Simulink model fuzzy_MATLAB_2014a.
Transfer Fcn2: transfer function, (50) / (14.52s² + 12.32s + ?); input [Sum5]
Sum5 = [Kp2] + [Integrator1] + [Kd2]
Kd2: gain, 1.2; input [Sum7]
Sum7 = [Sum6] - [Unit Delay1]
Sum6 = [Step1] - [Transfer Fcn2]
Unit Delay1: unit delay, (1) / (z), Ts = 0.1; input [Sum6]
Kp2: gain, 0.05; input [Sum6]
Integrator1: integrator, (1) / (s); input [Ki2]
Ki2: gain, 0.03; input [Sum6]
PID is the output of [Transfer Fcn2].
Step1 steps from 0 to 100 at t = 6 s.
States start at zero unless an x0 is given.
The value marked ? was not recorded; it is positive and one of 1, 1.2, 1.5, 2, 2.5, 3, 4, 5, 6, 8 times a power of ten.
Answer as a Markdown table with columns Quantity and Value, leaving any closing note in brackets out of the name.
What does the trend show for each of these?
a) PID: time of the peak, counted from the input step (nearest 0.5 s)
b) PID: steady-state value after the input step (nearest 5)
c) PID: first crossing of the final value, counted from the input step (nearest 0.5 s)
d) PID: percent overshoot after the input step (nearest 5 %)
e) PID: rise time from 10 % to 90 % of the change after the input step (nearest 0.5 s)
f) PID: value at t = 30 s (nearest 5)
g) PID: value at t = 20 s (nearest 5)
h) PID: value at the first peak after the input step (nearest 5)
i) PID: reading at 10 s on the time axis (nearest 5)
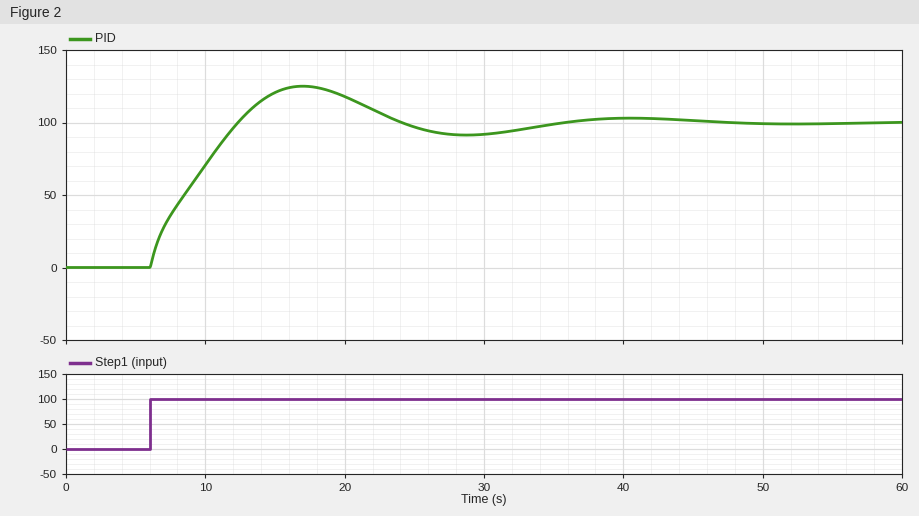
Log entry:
| Quantity | Value |
|---|---|
| PID: time of the peak, counted from the input step | 11.0 s |
| PID: steady-state value after the input step | 100 |
| PID: first crossing of the final value, counted from the input step | 6.5 s |
| PID: percent overshoot after the input step | 25 % |
| PID: rise time from 10 % to 90 % of the change after the input step | 5.0 s |
| PID: value at t = 30 s | 90 |
| PID: value at t = 20 s | 120 |
| PID: value at the first peak after the input step | 125 |
| PID: reading at 10 s on the time axis | 70 |
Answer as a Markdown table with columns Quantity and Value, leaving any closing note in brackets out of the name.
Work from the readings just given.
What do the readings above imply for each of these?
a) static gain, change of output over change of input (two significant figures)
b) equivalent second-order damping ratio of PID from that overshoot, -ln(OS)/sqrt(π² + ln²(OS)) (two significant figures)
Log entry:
| Quantity | Value |
|---|---|
| static gain, change of output over change of input | 1.0 |
| equivalent second-order damping ratio of PID from that overshoot, -ln(OS)/sqrt(π² + ln²(OS)) | 0.40 |
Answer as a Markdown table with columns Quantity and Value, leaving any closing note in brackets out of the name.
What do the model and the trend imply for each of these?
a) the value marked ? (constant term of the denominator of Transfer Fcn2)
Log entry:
| Quantity | Value |
|---|---|
| the value marked ? | 2 |
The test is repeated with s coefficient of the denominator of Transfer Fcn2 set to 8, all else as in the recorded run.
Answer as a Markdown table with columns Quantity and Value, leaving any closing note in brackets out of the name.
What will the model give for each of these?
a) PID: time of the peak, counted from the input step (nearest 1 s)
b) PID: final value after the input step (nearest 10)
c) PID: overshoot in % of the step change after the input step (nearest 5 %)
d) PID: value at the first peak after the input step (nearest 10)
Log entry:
| Quantity | Value |
|---|---|
| PID: time of the peak, counted from the input step | 10 s |
| PID: final value after the input step | 100 |
| PID: overshoot in % of the step change after the input step | 20 % |
| PID: value at the first peak after the input step | 120 |
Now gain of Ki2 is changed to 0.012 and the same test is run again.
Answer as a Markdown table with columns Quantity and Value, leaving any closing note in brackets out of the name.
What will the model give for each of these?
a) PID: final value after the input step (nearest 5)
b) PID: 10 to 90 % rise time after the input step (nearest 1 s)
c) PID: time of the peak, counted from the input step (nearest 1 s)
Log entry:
| Quantity | Value |
|---|---|
| PID: final value after the input step | 100 |
| PID: 10 to 90 % rise time after the input step | 9 s |
| PID: time of the peak, counted from the input step | 19 s |
